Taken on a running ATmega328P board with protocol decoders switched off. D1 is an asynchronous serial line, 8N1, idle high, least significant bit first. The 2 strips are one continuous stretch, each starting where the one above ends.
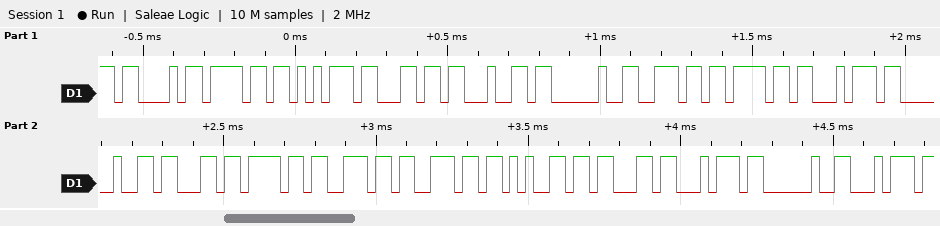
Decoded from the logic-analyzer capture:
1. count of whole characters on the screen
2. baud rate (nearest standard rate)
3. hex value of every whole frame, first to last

19
38400 baud
43 6F 75 6C 64 20 6E 6F 74 20 63 6F 6E 6E 65 63 74 20 74
